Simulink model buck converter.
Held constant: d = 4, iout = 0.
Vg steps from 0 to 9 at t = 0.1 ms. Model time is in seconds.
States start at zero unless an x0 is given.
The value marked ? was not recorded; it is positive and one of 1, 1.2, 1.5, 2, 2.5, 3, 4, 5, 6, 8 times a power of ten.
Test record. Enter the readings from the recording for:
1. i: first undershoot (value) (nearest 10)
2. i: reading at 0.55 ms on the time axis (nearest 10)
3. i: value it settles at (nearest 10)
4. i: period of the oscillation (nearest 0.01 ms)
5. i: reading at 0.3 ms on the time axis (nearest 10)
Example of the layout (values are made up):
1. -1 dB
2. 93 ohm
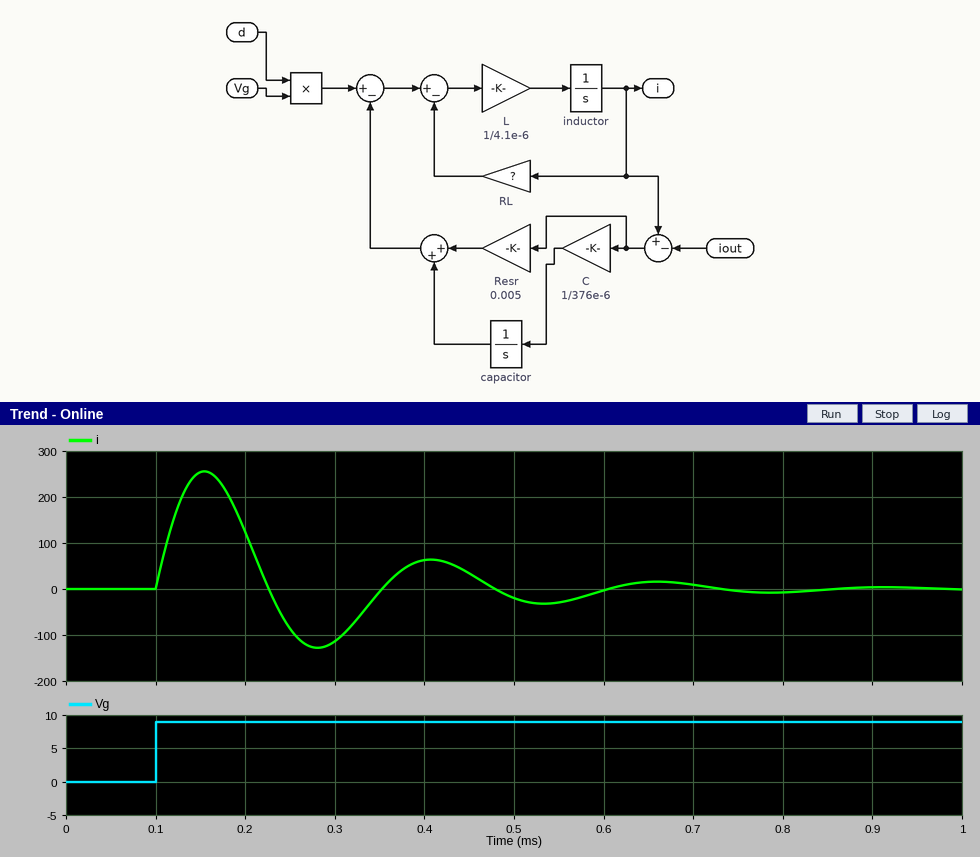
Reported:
1. -130
2. -30
3. 0
4. 0.25 ms
5. -110
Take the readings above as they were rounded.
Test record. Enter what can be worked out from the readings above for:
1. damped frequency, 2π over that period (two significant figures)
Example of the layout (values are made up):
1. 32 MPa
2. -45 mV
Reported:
1. 25 rad/ms
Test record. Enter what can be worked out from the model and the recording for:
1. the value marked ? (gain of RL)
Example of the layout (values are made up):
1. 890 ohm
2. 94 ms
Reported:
1. 0.04
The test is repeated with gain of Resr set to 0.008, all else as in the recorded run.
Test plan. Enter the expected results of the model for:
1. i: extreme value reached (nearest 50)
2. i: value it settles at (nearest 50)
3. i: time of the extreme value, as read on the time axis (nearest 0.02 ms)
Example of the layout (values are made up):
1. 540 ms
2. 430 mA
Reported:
1. 250
2. 0
3. 0.16 ms
